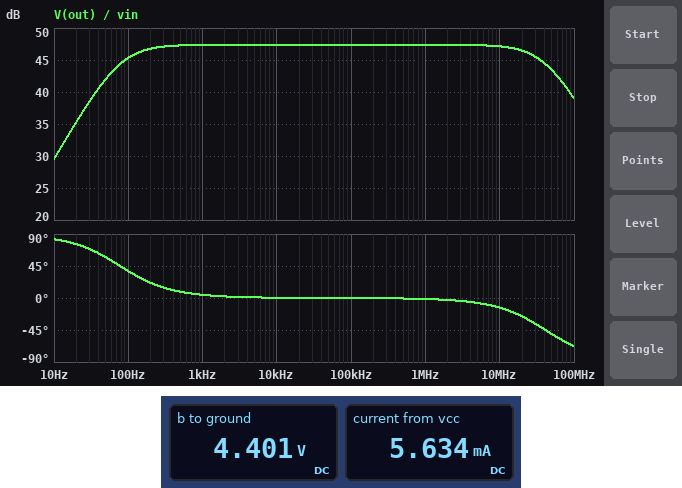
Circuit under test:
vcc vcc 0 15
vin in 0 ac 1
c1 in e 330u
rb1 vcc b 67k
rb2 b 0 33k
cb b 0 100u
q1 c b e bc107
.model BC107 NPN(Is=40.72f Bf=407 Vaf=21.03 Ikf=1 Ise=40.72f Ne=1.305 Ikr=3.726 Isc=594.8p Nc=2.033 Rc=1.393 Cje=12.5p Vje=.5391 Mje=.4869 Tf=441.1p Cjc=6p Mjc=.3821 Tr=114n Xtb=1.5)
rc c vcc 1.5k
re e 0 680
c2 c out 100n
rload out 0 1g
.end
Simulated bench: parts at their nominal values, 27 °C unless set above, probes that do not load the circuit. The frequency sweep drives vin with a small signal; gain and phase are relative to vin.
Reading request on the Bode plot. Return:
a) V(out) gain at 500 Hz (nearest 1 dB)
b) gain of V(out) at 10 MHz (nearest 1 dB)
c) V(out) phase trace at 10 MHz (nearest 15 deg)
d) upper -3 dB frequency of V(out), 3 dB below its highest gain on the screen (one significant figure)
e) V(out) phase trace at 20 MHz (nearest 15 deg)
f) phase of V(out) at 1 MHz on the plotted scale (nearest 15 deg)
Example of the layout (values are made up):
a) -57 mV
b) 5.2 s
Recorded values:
a) 47 dB
b) 47 dB
c) -15 deg
d) 40 MHz
e) -30 deg
f) 0 deg
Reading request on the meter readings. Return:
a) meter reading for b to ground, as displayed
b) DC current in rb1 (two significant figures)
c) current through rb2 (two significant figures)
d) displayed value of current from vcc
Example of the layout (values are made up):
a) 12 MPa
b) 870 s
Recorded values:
a) 4.401 V
b) 160 µA
c) 130 µA
d) 5.634 mA
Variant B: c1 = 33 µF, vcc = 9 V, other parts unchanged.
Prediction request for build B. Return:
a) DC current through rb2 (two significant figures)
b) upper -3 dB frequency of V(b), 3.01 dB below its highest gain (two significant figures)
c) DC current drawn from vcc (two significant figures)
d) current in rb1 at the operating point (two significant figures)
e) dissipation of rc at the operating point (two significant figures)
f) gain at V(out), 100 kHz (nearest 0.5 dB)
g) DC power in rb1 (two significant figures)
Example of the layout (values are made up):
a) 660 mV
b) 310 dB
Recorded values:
a) 80 µA
b) 470 Hz
c) 3.0 mA
d) 95 µA
e) 13 mW
f) 43.0 dB
g) 600 µW
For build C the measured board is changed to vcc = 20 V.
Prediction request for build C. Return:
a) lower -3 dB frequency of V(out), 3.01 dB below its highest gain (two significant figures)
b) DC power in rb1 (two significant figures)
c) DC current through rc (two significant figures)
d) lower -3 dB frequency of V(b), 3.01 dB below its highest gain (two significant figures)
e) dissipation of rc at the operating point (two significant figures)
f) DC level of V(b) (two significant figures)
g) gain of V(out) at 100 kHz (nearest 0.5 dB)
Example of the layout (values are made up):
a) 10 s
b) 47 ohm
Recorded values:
a) 98 Hz
b) 3.0 mW
c) 7.6 mA
d) 85 mHz
e) 87 mW
f) 5.9 V
g) 49.5 dB
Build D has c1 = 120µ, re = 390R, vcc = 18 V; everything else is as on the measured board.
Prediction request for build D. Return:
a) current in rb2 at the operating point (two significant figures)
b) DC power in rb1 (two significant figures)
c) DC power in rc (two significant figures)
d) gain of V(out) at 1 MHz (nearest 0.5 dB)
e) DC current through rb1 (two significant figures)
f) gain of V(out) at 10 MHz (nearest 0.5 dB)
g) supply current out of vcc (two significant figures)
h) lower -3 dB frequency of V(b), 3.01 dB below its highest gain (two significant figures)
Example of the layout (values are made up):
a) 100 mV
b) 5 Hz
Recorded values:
a) 130 µA
b) 2.8 mW
c) 130 mW
d) 43.0 dB
e) 200 µA
f) 36.5 dB
g) 9.6 mA
h) 1.7 Hz
